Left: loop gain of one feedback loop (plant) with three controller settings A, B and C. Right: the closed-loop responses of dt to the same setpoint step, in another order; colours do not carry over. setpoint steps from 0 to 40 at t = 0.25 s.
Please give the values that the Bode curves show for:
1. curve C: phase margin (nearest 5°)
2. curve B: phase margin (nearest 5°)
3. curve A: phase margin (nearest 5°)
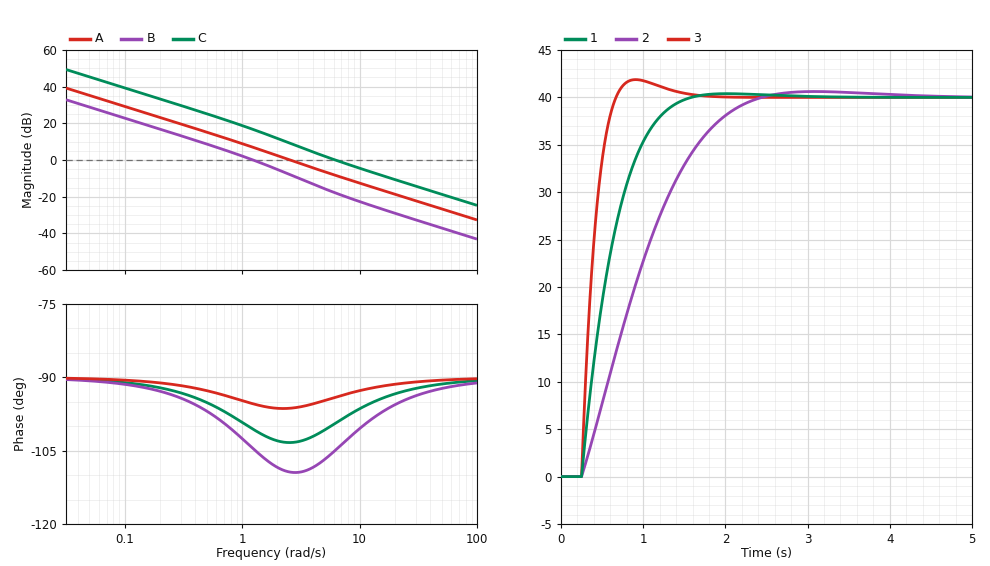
80°
75°
85°
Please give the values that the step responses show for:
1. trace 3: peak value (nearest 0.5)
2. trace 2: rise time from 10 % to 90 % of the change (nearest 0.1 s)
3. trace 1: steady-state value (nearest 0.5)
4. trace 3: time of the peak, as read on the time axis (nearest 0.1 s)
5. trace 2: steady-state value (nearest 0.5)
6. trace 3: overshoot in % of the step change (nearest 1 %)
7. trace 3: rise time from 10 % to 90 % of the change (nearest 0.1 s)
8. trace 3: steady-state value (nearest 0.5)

42.0
1.4 s
40.0
0.9 s
40.0
5 %
0.3 s
40.0
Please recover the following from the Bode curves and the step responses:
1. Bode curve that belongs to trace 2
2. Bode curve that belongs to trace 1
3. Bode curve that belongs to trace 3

B
A
C
